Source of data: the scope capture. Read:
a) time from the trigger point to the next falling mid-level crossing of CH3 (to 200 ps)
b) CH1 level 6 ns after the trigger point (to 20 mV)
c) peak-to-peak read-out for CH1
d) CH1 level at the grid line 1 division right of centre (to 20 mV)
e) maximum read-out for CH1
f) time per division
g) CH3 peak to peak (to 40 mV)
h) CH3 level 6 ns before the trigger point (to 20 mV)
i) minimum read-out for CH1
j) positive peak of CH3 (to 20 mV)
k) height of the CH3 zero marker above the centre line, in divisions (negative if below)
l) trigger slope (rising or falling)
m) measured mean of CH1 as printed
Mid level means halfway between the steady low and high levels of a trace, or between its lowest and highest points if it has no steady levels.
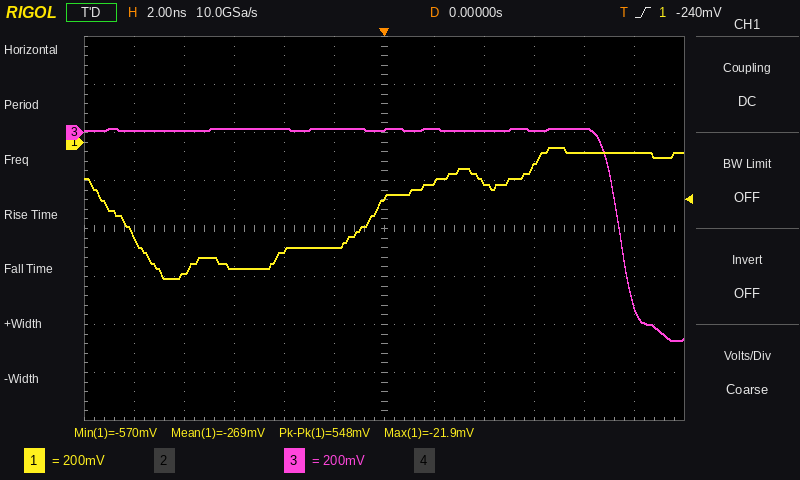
9.4 ns
-100 mV
548 mV
-160 mV
-21.9 mV
2 ns
880 mV
20 mV
-570 mV
20 mV
+2.0 div
rising
-269 mV
